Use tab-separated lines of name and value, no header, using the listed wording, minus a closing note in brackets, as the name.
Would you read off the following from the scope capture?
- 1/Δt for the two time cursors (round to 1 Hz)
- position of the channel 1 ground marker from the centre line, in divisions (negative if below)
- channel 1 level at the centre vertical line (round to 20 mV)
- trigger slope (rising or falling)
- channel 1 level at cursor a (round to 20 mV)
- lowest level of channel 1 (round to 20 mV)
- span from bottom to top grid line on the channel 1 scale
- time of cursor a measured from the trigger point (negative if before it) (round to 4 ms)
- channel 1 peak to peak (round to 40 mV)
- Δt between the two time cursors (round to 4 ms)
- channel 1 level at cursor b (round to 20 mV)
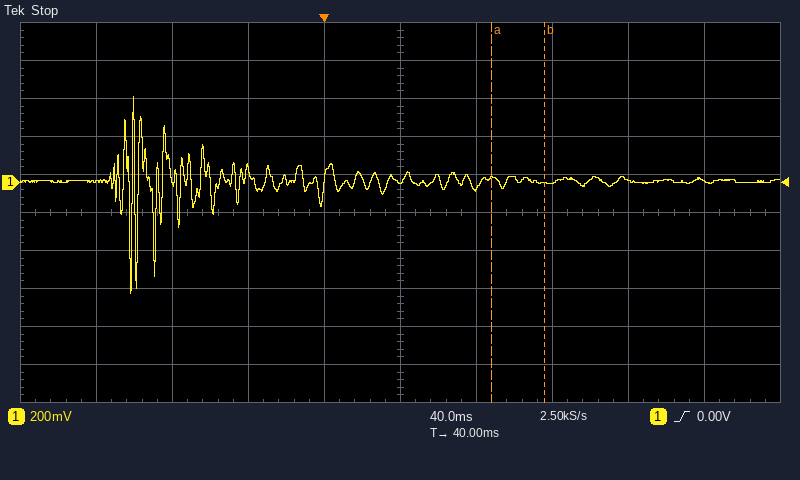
1/Δt for the two time cursors	36 Hz
position of the channel 1 ground marker from the centre line, in divisions	+0.8 div
channel 1 level at the centre vertical line	0 mV
trigger slope	rising
channel 1 level at cursor a	20 mV
lowest level of channel 1	-580 mV
span from bottom to top grid line on the channel 1 scale	2 V
time of cursor a measured from the trigger point (negative if before it)	+88 ms
channel 1 peak to peak	1.04 V
Δt between the two time cursors	28 ms
channel 1 level at cursor b	0 mV
